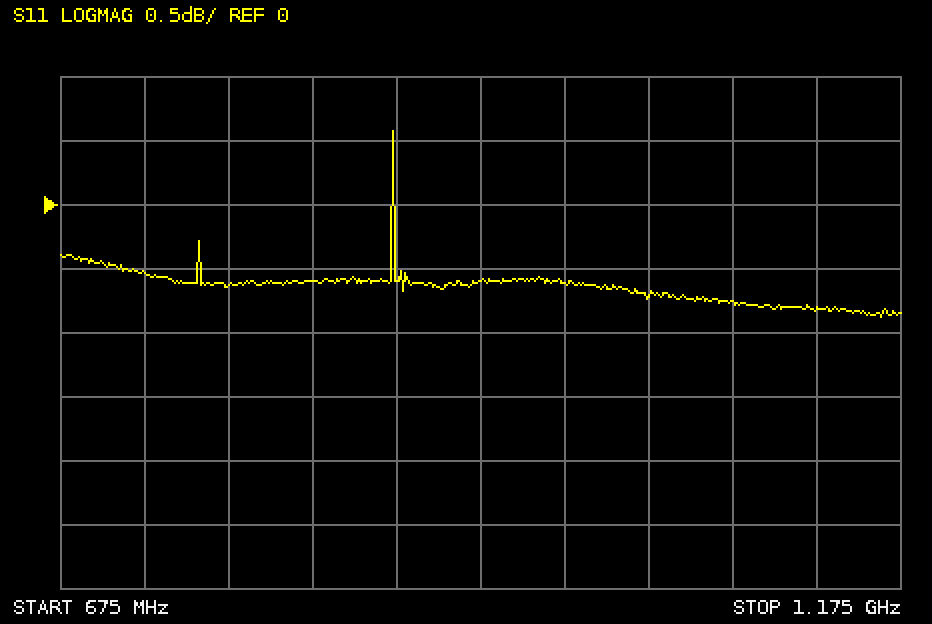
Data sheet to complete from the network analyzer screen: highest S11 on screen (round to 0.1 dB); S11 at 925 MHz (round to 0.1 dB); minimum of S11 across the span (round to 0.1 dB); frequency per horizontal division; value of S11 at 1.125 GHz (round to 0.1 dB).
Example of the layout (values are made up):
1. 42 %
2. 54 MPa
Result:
1. 0.6 dB
2. -0.6 dB
3. -0.9 dB
4. 50 MHz
5. -0.8 dB
